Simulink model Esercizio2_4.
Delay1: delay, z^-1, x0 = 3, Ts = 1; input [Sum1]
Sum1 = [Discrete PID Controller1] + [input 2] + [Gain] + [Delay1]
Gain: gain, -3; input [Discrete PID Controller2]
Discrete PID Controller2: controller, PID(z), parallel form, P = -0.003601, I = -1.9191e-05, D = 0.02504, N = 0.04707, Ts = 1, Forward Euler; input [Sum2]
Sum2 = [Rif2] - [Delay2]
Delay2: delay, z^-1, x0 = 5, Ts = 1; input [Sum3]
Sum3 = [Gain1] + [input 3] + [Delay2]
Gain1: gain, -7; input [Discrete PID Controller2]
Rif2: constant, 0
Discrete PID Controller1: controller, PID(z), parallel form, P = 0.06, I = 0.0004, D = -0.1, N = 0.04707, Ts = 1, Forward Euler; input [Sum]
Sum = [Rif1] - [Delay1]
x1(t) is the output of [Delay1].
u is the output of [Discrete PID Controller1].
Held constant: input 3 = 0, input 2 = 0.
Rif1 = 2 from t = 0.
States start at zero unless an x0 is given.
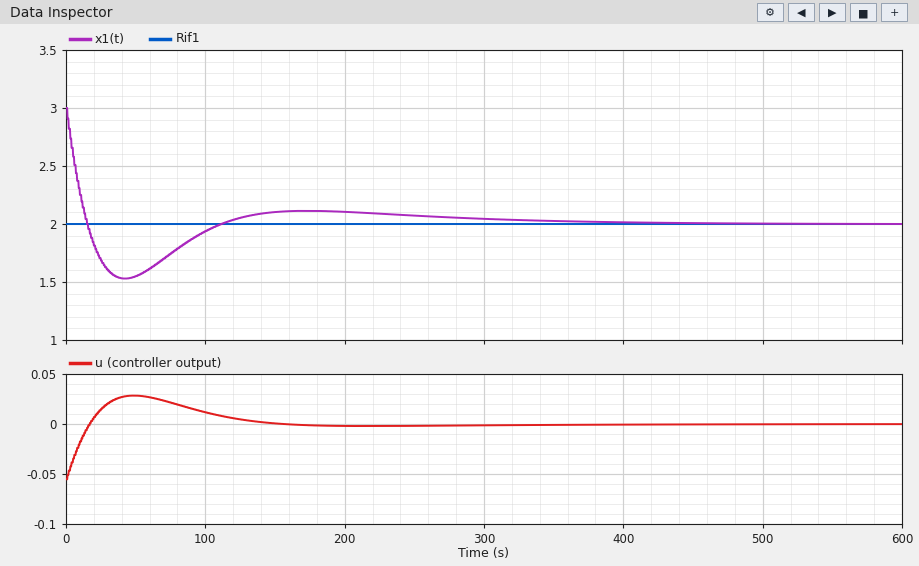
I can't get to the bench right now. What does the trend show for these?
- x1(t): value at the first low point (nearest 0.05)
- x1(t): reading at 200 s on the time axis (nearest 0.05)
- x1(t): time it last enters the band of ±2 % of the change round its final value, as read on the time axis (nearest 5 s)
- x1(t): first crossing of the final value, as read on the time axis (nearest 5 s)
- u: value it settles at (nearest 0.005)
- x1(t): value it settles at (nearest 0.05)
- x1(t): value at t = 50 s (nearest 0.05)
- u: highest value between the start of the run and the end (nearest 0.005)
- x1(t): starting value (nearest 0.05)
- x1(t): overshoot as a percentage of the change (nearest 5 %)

1.55
2.10
375 s
15 s
0.000
2.00
1.55
0.030
3.00
45 %
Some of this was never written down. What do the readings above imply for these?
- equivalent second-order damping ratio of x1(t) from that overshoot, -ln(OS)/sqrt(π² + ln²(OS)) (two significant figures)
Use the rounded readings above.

0.25
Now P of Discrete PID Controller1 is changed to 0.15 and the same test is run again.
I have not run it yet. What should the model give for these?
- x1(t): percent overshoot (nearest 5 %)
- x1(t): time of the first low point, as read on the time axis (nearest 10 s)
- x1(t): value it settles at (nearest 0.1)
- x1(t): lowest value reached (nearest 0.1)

25 %
30 s
2.0
1.8
